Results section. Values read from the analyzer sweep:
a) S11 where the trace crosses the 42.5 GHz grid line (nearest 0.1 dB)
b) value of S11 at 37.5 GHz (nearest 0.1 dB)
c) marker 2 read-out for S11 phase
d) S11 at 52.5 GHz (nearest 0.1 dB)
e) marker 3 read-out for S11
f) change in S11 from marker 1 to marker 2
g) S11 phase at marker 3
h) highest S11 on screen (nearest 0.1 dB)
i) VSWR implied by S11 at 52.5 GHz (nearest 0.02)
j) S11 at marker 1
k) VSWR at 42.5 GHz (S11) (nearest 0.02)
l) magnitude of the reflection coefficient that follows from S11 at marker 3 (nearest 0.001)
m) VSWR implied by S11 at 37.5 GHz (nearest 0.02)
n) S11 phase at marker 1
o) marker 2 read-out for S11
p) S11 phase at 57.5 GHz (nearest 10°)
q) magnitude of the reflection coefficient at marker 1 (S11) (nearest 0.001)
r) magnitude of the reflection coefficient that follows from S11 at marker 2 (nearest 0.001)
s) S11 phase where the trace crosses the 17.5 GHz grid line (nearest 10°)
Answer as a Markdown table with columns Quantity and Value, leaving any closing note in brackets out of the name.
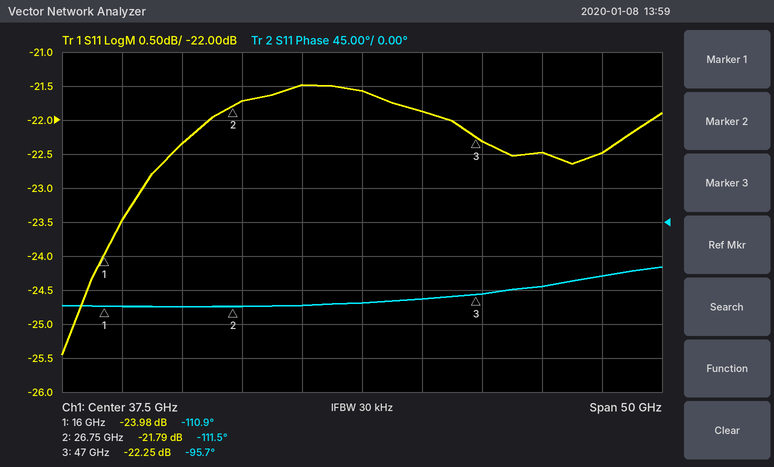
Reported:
| Quantity | Value |
|---|---|
| S11 where the trace crosses the 42.5 GHz grid line | -21.9 dB |
| value of S11 at 37.5 GHz | -21.6 dB |
| marker 2 read-out for S11 phase | -111.5° |
| S11 at 52.5 GHz | -22.5 dB |
| marker 3 read-out for S11 | -22.25 dB |
| change in S11 from marker 1 to marker 2 | 2.19 dB |
| S11 phase at marker 3 | -95.7° |
| highest S11 on screen | -21.5 dB |
| VSWR implied by S11 at 52.5 GHz | 1.16 |
| S11 at marker 1 | -23.98 dB |
| VSWR at 42.5 GHz (S11) | 1.18 |
| magnitude of the reflection coefficient that follows from S11 at marker 3 | 0.077 |
| VSWR implied by S11 at 37.5 GHz | 1.18 |
| S11 phase at marker 1 | -110.9° |
| marker 2 read-out for S11 | -21.79 dB |
| S11 phase at 57.5 GHz | -70° |
| magnitude of the reflection coefficient at marker 1 (S11) | 0.063 |
| magnitude of the reflection coefficient that follows from S11 at marker 2 | 0.081 |
| S11 phase where the trace crosses the 17.5 GHz grid line | -110° |
